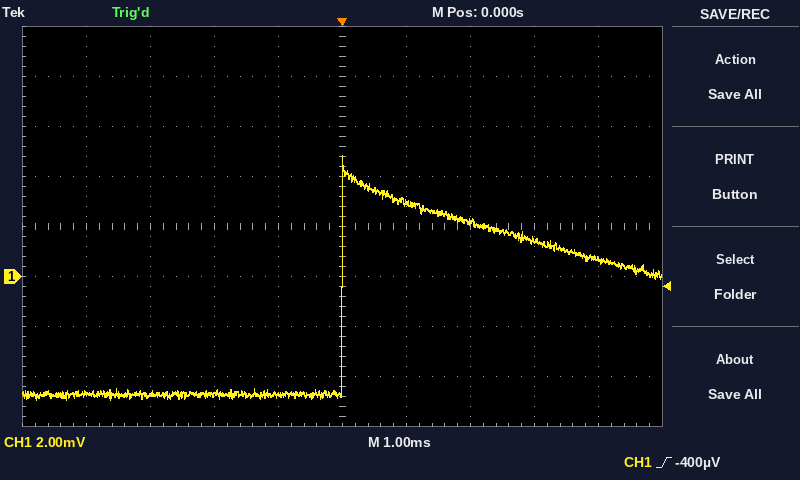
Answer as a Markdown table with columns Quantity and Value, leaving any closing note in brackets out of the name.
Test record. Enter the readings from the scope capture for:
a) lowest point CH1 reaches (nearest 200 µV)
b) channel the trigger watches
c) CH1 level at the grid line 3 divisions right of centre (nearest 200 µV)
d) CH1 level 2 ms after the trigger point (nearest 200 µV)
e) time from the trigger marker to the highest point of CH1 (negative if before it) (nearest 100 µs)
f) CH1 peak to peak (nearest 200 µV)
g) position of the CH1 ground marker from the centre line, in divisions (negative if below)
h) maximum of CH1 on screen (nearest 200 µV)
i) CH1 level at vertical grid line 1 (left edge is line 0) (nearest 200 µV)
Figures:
| Quantity | Value |
|---|---|
| lowest point CH1 reaches | -5.0 mV |
| channel the trigger watches | CH1 |
| CH1 level at the grid line 3 divisions right of centre | 1.4 mV |
| CH1 level 2 ms after the trigger point | 2.2 mV |
| time from the trigger marker to the highest point of CH1 (negative if before it) | 0.0 ms |
| CH1 peak to peak | 9.8 mV |
| position of the CH1 ground marker from the centre line, in divisions | -1.0 div |
| maximum of CH1 on screen | 4.8 mV |
| CH1 level at vertical grid line 1 (left edge is line 0) | -4.6 mV |
